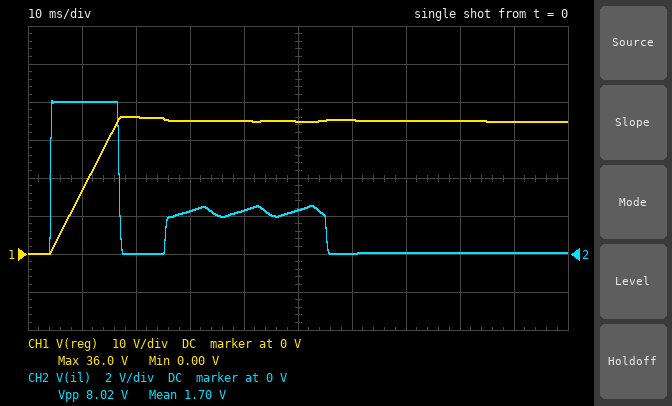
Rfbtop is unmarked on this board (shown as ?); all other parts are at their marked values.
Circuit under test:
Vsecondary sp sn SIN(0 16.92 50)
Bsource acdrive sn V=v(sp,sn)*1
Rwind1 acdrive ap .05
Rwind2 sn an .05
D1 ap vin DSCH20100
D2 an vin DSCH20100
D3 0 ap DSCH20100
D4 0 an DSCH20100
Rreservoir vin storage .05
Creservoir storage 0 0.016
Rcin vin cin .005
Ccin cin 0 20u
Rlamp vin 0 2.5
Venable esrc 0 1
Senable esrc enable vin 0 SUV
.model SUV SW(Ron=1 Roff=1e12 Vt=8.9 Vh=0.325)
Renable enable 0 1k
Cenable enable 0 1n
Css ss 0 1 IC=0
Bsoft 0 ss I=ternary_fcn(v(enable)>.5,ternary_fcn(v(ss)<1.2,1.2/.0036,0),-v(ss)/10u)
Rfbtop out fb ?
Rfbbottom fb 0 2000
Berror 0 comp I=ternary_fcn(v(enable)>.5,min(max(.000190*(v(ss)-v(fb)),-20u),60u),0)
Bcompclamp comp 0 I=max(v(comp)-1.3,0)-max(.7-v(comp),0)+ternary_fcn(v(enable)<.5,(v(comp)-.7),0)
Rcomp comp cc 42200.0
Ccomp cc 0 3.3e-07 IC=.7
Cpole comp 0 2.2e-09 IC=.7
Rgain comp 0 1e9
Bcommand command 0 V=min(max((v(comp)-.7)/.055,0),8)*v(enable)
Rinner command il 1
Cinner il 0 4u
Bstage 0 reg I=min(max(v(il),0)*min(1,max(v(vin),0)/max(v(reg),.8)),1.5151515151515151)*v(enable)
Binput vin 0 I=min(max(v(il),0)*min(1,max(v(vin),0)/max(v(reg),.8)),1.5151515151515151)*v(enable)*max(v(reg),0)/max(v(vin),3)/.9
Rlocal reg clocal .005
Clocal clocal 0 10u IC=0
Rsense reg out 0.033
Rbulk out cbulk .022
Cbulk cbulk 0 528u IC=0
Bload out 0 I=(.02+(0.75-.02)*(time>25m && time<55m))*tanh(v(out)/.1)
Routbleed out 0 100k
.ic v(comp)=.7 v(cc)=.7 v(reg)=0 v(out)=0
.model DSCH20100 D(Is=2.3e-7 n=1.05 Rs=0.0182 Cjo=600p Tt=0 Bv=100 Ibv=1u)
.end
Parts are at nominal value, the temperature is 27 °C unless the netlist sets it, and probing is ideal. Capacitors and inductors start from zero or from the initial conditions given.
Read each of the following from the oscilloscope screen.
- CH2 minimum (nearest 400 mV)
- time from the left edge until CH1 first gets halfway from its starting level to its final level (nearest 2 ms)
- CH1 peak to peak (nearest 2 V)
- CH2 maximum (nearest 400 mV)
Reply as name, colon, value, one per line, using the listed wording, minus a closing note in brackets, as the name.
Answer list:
CH2 minimum: 0 V
time from the left edge until CH1 first gets halfway from its starting level to its final level: 10 ms
CH1 peak to peak: 36 V
CH2 maximum: 8.0 V
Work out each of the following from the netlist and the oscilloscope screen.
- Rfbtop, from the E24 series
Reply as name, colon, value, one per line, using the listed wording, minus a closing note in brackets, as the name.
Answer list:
Rfbtop, from the E24 series: 56 kΩ
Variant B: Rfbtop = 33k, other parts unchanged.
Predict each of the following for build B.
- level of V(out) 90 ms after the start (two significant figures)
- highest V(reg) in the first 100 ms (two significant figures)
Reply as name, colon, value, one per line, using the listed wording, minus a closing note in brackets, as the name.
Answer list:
level of V(out) 90 ms after the start: 21 V
highest V(reg) in the first 100 ms: 22 V
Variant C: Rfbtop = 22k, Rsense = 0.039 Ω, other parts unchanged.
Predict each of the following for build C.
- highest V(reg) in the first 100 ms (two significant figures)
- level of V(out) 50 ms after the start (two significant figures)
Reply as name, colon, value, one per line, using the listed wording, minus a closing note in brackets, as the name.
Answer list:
highest V(reg) in the first 100 ms: 15 V
level of V(out) 50 ms after the start: 14 V
